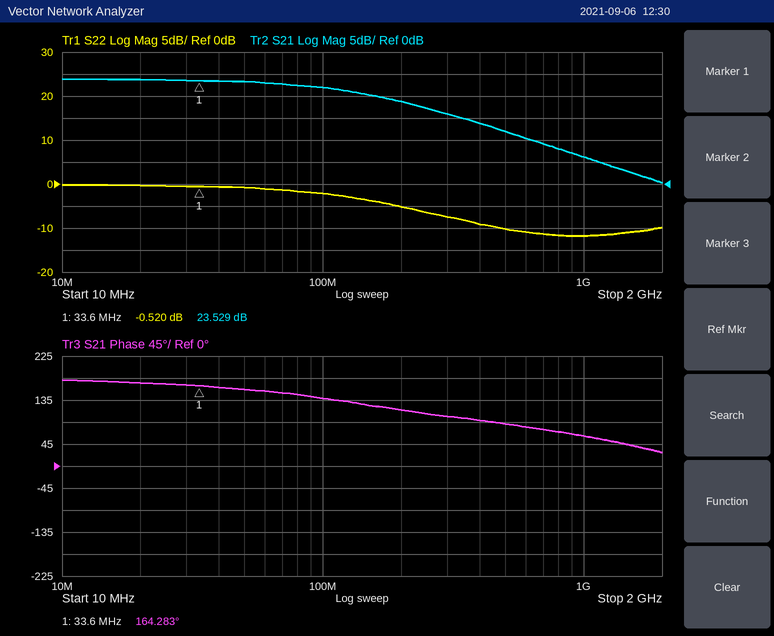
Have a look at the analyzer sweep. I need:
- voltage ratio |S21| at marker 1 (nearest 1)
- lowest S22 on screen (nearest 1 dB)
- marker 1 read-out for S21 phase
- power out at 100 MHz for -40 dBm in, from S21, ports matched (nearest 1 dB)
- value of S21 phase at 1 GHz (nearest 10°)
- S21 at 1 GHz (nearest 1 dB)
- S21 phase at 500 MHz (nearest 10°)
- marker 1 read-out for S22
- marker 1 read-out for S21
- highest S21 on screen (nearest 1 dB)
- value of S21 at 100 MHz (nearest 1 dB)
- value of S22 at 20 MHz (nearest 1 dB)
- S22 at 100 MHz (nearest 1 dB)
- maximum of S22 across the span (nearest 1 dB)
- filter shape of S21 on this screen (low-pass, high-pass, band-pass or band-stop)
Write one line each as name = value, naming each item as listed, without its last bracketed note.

voltage ratio |S21| at marker 1 = 15
lowest S22 on screen = -12 dB
marker 1 read-out for S21 phase = 164.283°
power out at 100 MHz for -40 dBm in, from S21, ports matched = -18 dBm
value of S21 phase at 1 GHz = 60°
S21 at 1 GHz = 6 dB
S21 phase at 500 MHz = 90°
marker 1 read-out for S22 = -0.520 dB
marker 1 read-out for S21 = 23.529 dB
highest S21 on screen = 24 dB
value of S21 at 100 MHz = 22 dB
value of S22 at 20 MHz = 0 dB
S22 at 100 MHz = -2 dB
maximum of S22 across the span = 0 dB
filter shape of S21 on this screen = low-pass
